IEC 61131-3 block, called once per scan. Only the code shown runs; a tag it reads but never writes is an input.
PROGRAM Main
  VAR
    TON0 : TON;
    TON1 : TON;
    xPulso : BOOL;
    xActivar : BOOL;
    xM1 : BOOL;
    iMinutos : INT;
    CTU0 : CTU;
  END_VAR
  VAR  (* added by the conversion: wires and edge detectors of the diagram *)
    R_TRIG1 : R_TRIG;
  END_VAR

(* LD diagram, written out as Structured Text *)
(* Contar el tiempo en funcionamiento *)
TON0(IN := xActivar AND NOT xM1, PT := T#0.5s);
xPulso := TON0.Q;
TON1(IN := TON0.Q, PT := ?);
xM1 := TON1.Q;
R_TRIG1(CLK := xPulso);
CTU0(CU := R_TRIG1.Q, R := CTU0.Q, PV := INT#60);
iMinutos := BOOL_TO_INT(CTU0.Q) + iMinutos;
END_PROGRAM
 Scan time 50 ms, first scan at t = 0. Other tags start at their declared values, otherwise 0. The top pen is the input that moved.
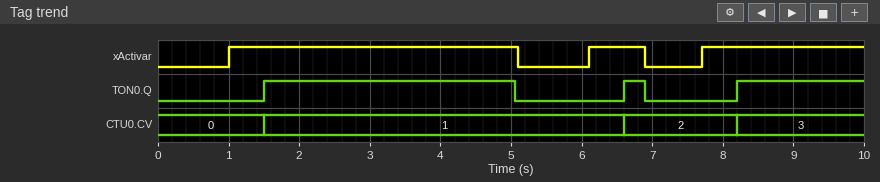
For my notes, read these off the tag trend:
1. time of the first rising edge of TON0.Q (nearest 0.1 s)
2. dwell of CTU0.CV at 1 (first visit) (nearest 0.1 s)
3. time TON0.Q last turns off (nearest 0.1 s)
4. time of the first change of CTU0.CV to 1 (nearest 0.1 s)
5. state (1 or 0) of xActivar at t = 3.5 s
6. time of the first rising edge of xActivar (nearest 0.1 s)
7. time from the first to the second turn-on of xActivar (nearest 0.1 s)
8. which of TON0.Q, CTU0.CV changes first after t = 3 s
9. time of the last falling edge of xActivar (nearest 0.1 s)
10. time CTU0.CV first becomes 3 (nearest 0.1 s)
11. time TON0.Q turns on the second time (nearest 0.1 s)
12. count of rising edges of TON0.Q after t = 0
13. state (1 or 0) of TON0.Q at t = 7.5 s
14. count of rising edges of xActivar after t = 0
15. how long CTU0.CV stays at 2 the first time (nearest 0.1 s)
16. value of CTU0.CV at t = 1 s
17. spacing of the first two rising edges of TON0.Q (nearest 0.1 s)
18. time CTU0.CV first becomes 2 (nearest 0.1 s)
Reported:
1.5 s
5.1 s
6.9 s
1.5 s
1
1.0 s
5.1 s
TON0.Q
6.9 s
8.2 s
6.6 s
3
0
3
1.6 s
0
5.1 s
6.6 s
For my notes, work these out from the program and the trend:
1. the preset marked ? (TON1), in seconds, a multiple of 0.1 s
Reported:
3.5 s
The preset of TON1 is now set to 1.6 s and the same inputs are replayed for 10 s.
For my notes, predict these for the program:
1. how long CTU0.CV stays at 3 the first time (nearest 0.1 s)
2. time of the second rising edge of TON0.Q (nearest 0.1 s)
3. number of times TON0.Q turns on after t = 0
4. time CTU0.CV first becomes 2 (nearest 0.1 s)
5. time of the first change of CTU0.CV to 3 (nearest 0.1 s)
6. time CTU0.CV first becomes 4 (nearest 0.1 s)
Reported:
1.6 s
3.7 s
4
3.7 s
6.6 s
8.2 s
